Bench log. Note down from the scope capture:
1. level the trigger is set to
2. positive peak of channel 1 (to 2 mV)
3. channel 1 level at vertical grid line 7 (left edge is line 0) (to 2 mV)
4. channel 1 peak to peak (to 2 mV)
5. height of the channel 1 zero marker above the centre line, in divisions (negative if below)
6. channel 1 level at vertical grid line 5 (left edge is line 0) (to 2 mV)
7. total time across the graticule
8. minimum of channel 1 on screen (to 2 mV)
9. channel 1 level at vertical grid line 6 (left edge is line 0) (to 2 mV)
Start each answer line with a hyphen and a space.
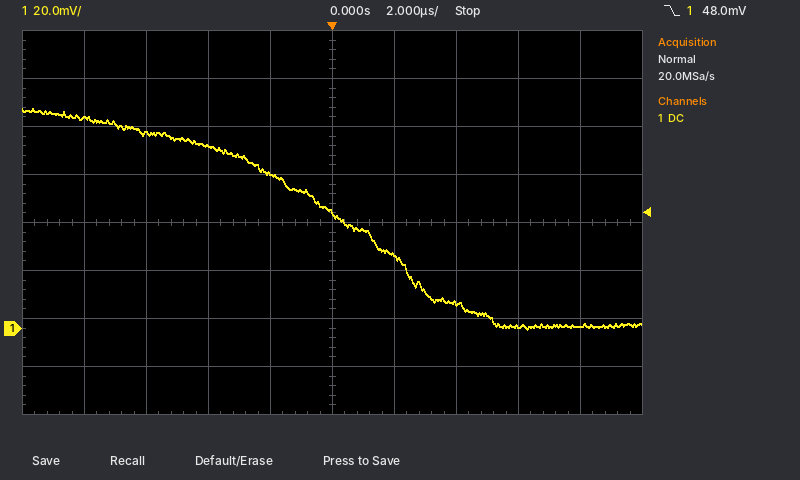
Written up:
- 48.0 mV
- 92 mV
- 10 mV
- 92 mV
- -2.2 div
- 48 mV
- 20 µs
- 0 mV
- 30 mV
